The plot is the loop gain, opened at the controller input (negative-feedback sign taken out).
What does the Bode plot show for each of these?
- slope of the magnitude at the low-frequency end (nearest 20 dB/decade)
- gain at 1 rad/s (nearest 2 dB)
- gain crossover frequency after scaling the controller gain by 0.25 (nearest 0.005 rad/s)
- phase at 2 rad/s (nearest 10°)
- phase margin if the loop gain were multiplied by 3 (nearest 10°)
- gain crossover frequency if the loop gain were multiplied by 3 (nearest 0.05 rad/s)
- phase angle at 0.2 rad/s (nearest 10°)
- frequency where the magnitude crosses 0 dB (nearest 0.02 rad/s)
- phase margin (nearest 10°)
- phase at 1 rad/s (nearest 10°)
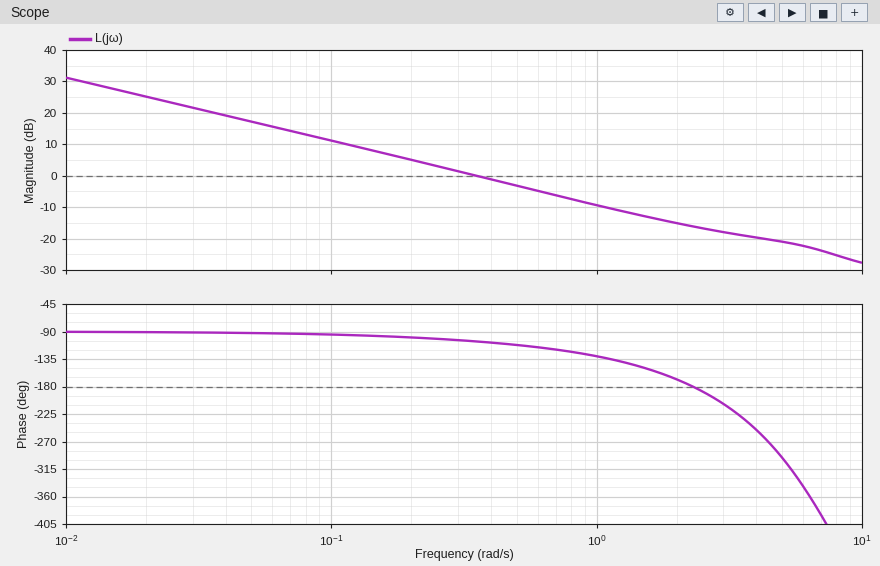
-20 dB/decade
-10 dB
0.090 rad/s
-170°
50°
1.00 rad/s
-100°
0.36 rad/s
70°
-130°
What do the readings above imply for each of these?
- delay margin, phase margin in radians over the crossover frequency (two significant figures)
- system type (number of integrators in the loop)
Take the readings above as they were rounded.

3.4 s
1
